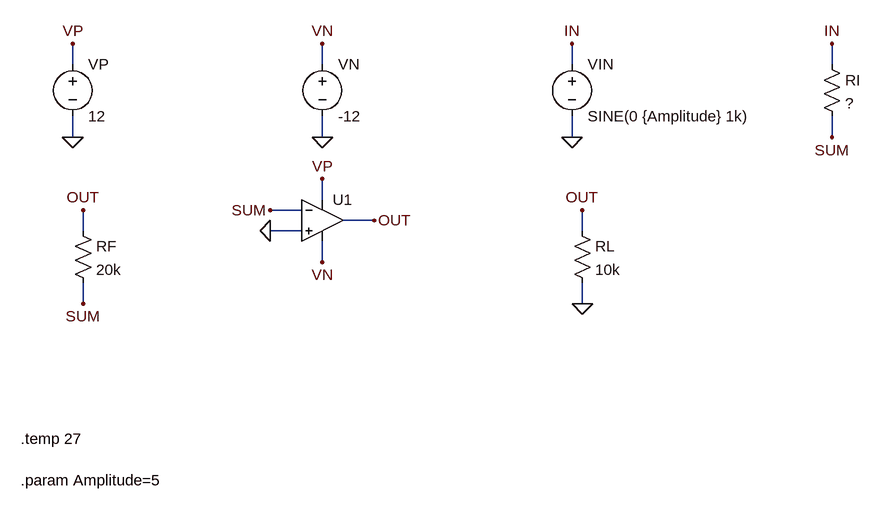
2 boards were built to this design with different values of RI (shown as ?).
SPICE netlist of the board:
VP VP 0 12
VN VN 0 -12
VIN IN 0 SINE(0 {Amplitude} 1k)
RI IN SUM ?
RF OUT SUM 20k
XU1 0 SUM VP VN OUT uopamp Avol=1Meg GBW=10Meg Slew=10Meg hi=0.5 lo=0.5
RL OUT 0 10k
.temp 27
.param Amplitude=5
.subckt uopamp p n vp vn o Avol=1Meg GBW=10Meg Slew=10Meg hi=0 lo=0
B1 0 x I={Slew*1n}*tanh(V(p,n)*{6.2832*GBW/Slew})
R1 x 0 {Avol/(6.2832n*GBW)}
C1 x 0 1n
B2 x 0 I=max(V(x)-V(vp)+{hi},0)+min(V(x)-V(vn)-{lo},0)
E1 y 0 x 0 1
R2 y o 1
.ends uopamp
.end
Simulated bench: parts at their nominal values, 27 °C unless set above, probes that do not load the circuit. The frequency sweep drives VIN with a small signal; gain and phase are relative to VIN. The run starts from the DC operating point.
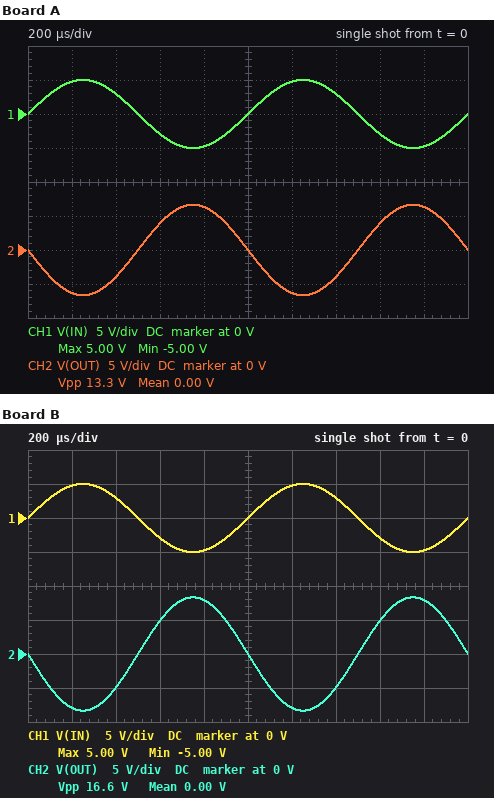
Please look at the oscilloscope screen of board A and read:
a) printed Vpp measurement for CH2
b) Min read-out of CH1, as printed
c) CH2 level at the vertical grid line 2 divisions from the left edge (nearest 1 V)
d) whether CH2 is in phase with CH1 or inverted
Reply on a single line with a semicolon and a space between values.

13.3 V; -5.00 V; -4 V; inverted
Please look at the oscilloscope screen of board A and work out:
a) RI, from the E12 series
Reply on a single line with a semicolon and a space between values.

15 kΩ
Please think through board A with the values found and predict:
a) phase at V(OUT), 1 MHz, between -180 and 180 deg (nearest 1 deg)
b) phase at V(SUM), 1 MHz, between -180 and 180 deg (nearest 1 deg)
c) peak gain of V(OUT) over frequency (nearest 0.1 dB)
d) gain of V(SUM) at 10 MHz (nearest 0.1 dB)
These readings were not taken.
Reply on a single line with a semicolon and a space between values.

167 deg; 77 deg; 2.5 dB; -5.6 dB
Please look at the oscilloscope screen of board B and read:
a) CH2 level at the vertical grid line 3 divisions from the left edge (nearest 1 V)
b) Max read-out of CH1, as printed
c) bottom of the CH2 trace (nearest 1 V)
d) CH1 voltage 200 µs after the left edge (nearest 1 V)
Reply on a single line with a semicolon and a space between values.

5 V; 5.00 V; -8 V; 5 V
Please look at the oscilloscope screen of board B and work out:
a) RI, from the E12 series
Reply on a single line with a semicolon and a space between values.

12 kΩ
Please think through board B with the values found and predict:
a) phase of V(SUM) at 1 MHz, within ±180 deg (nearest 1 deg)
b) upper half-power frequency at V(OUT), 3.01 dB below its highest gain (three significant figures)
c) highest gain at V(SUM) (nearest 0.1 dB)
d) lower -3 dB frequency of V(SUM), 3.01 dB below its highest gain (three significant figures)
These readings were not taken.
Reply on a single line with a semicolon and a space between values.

75 deg; 3.75 MHz; -4.1 dB; 3.75 MHz
